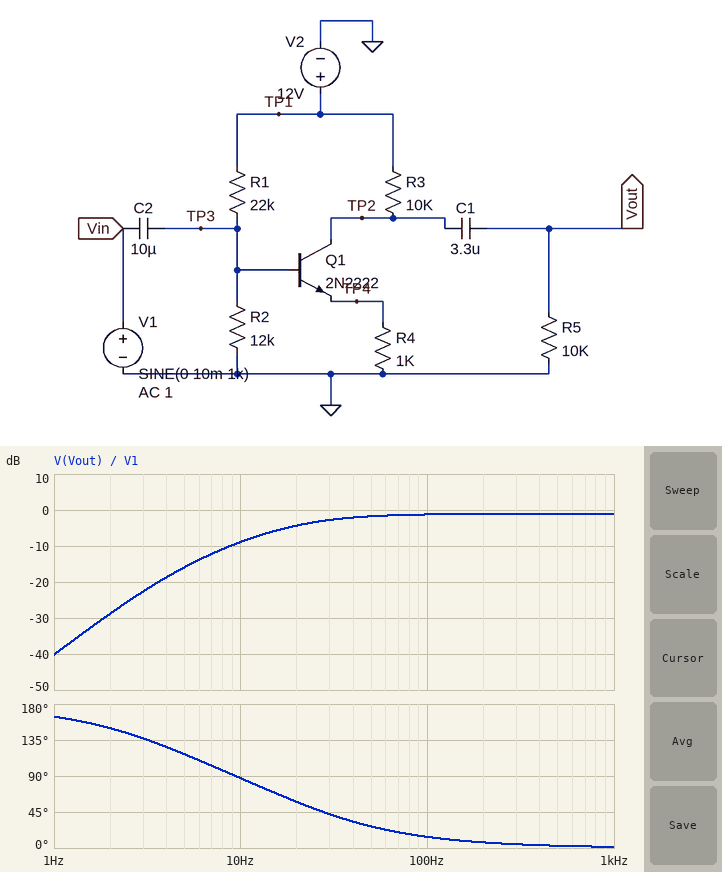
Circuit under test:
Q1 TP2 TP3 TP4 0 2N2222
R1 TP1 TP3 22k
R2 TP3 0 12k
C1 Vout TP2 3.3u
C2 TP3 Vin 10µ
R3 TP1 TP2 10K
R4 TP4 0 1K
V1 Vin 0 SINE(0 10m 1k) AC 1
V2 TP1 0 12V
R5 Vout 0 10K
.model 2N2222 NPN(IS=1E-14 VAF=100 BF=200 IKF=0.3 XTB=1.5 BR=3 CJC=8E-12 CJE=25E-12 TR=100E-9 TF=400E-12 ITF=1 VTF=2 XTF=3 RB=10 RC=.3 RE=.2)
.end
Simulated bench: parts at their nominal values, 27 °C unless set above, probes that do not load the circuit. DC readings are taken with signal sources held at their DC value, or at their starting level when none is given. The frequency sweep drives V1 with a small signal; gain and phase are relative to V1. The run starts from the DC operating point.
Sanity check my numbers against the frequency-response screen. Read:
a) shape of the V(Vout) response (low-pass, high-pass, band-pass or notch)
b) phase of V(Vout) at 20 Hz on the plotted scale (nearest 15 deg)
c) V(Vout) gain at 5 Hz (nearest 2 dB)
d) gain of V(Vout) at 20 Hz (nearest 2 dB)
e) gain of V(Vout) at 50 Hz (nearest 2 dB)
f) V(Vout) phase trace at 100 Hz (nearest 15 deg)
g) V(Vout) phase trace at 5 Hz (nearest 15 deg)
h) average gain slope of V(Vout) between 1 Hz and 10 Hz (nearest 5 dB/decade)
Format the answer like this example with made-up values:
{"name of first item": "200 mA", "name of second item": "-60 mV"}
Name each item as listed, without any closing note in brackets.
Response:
{"shape of the V(Vout) response": "high-pass", "phase of V(Vout) at 20 Hz on the plotted scale": "60 deg", "V(Vout) gain at 5 Hz": "-16 dB", "gain of V(Vout) at 20 Hz": "-4 dB", "gain of V(Vout) at 50 Hz": "-2 dB", "V(Vout) phase trace at 100 Hz": "15 deg", "V(Vout) phase trace at 5 Hz": "120 deg", "average gain slope of V(Vout) between 1 Hz and 10 Hz": "30 dB/decade"}
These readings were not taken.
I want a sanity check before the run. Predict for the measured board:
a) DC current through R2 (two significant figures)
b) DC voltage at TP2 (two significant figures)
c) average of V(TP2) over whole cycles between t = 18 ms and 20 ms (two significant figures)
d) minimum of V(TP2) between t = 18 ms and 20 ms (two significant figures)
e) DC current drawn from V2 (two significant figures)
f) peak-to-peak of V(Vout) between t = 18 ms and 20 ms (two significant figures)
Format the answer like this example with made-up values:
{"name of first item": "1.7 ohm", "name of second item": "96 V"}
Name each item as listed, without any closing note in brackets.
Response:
{"DC current through R2": "170 µA", "DC voltage at TP2": "1.4 V", "average of V(TP2) over whole cycles between t = 18 ms and 20 ms": "1.4 V", "minimum of V(TP2) between t = 18 ms and 20 ms": "1.4 V", "DC current drawn from V2": "1.5 mA", "peak-to-peak of V(Vout) between t = 18 ms and 20 ms": "18 mV"}
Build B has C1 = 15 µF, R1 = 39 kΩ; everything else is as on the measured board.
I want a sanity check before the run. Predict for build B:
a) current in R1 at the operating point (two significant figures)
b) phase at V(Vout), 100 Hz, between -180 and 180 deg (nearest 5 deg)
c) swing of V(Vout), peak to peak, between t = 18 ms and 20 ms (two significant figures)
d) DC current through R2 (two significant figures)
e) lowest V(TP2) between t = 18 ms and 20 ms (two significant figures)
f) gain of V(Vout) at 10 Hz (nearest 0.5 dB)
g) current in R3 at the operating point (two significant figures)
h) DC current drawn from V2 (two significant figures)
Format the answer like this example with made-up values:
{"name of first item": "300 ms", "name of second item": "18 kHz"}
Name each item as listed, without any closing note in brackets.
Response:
{"current in R1 at the operating point": "260 µA", "phase at V(Vout), 100 Hz, between -180 and 180 deg": "10 deg", "swing of V(Vout), peak to peak, between t = 18 ms and 20 ms": "14 mV", "DC current through R2": "150 µA", "lowest V(TP2) between t = 18 ms and 20 ms": "1.2 V", "gain of V(Vout) at 10 Hz": "-9.5 dB", "current in R3 at the operating point": "1.1 mA", "DC current drawn from V2": "1.3 mA"}
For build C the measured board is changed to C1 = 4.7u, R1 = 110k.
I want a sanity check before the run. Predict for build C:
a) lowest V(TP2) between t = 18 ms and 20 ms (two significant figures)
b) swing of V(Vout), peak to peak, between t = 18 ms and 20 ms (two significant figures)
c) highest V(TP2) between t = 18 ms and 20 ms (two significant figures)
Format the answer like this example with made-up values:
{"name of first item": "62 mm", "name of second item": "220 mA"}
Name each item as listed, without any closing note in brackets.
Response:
{"lowest V(TP2) between t = 18 ms and 20 ms": "6.8 V", "swing of V(Vout), peak to peak, between t = 18 ms and 20 ms": "95 mV", "highest V(TP2) between t = 18 ms and 20 ms": "6.9 V"}
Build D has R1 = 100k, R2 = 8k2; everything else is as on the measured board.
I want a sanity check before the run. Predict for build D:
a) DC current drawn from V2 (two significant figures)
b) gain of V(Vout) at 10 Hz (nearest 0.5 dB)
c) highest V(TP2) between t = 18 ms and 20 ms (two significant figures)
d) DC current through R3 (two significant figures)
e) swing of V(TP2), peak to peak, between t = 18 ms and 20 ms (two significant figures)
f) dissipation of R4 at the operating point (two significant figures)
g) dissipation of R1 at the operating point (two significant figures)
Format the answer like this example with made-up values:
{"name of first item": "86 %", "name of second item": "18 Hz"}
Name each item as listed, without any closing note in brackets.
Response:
{"DC current drawn from V2": "390 µA", "gain of V(Vout) at 10 Hz": "12.5 dB", "highest V(TP2) between t = 18 ms and 20 ms": "9.3 V", "DC current through R3": "280 µA", "swing of V(TP2), peak to peak, between t = 18 ms and 20 ms": "91 mV", "dissipation of R4 at the operating point": "78 µW", "dissipation of R1 at the operating point": "1.2 mW"}
